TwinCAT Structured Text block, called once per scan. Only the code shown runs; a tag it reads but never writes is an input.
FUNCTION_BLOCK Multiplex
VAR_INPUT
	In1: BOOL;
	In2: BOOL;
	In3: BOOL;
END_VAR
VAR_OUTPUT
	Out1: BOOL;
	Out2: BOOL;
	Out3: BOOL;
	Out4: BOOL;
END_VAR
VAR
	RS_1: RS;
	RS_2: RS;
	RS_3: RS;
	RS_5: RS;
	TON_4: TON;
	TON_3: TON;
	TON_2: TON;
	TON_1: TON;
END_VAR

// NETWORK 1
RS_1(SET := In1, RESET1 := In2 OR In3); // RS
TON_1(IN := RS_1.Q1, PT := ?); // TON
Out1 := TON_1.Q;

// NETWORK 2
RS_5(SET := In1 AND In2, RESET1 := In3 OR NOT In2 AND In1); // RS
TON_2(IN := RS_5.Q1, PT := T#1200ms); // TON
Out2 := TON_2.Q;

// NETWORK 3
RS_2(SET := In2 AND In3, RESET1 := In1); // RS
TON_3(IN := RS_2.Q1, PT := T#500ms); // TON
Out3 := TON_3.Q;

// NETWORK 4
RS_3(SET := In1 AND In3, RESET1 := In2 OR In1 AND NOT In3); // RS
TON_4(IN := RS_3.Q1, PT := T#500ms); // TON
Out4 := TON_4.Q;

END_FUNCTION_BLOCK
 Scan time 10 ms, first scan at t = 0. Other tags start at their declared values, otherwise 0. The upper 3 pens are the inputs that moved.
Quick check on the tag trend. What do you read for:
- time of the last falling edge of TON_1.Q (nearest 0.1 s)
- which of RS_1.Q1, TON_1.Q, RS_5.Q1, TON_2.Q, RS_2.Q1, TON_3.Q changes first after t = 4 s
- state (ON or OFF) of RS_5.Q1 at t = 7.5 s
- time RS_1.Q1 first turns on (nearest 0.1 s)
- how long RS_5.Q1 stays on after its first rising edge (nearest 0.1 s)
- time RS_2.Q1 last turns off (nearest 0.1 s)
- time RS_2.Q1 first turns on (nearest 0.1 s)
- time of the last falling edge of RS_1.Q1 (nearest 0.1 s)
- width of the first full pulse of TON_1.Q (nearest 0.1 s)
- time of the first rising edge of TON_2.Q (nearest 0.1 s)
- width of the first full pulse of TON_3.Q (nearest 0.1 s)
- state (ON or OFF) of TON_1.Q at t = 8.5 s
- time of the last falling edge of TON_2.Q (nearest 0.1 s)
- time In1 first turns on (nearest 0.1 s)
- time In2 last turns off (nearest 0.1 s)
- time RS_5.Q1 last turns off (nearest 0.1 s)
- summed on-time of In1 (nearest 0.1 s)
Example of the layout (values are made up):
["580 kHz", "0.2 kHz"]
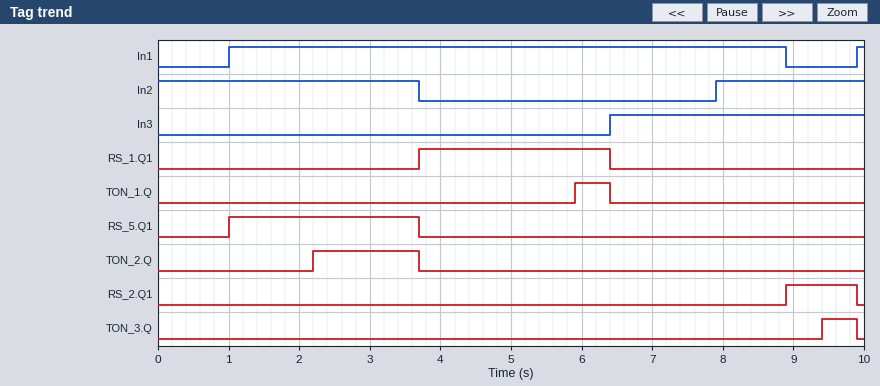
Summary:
["6.4 s", "TON_1.Q", "OFF", "3.7 s", "2.7 s", "9.9 s", "8.9 s", "6.4 s", "0.5 s", "2.2 s", "0.5 s", "OFF", "3.7 s", "1.0 s", "3.7 s", "3.7 s", "8.0 s"]
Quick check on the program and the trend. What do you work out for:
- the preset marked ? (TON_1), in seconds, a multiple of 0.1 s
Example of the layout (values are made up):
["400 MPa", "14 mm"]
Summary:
["2.2 s"]
